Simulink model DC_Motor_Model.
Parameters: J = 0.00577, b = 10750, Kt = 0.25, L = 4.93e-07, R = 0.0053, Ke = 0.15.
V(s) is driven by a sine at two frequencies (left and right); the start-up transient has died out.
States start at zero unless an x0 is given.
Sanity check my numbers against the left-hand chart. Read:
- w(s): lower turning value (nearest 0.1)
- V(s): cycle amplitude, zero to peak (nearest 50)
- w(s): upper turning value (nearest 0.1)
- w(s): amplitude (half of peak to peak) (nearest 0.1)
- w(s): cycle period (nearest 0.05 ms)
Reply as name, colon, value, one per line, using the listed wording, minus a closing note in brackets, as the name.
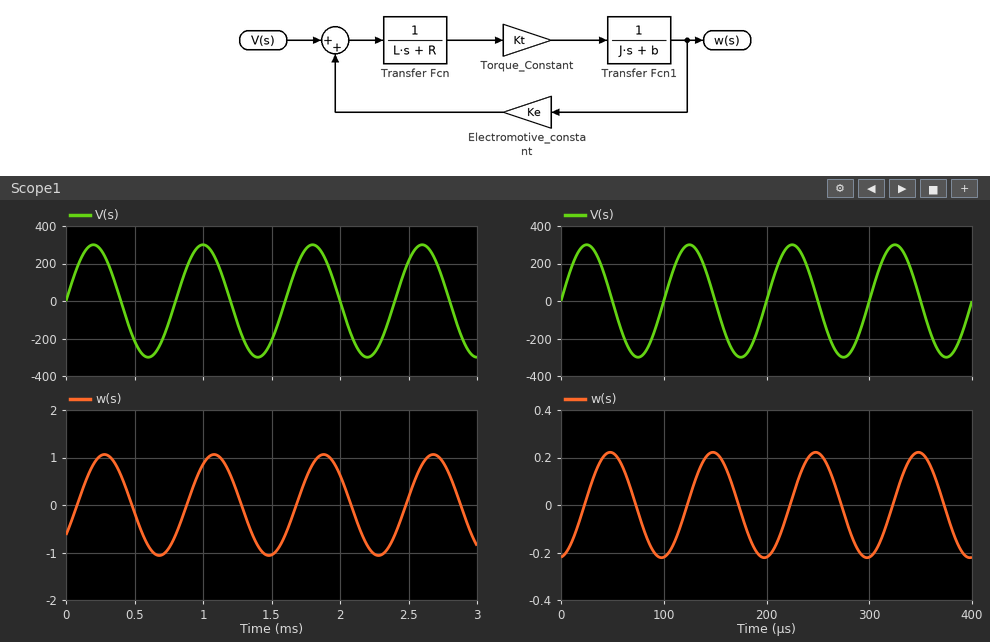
w(s): lower turning value: -1.1
V(s): cycle amplitude, zero to peak: 300
w(s): upper turning value: 1.1
w(s): amplitude (half of peak to peak): 1.1
w(s): cycle period: 0.80 ms
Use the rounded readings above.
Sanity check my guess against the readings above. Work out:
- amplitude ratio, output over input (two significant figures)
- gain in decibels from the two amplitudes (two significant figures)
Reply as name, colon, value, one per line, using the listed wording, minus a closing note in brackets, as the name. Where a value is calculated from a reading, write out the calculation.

amplitude ratio, output over input: 1.1 / 300 = 0.0037
gain in decibels from the two amplitudes: 20 log10(1.1 / 300) = -49 dB
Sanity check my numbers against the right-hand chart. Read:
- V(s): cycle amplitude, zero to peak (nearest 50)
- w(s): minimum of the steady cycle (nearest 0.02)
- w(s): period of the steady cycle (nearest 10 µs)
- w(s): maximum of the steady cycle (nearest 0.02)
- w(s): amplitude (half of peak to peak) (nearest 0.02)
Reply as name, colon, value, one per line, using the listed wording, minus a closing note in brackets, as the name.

V(s): cycle amplitude, zero to peak: 300
w(s): minimum of the steady cycle: -0.22
w(s): period of the steady cycle: 100 µs
w(s): maximum of the steady cycle: 0.22
w(s): amplitude (half of peak to peak): 0.22
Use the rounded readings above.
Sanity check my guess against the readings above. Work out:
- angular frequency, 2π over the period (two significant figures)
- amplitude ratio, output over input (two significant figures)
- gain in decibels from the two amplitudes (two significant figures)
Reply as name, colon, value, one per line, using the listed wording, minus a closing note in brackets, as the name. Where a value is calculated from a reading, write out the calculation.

angular frequency, 2π over the period: 2π / 100 = 0.063 rad/µs
amplitude ratio, output over input: 0.22 / 300 = 0.00073
gain in decibels from the two amplitudes: 20 log10(0.22 / 300) = -63 dB
